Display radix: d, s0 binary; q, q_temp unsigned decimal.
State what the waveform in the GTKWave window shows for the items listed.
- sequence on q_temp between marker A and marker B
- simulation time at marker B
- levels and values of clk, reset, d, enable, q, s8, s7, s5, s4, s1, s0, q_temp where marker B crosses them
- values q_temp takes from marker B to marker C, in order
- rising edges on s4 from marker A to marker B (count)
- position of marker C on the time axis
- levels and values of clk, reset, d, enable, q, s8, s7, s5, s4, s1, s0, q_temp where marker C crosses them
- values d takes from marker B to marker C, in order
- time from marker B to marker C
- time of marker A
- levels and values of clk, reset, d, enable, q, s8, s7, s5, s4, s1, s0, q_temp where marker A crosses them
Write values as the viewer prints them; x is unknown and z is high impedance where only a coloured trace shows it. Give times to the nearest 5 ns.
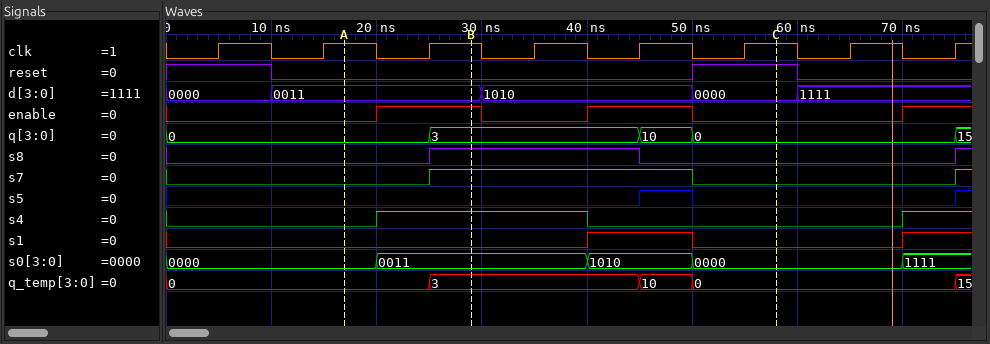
0, 3
30 ns
clk=1, reset=0, d=0011, enable=1, q=3, s8=1, s7=1, s5=0, s4=1, s1=0, s0=0011, q_temp=3
3, 10, 0
1
60 ns
clk=1, reset=1, d=0000, enable=0, q=0, s8=0, s7=0, s5=0, s4=0, s1=0, s0=0000, q_temp=0
0011, 1010, 0000
30 ns
15 ns
clk=1, reset=0, d=0011, enable=0, q=0, s8=0, s7=0, s5=0, s4=0, s1=0, s0=0000, q_temp=0
